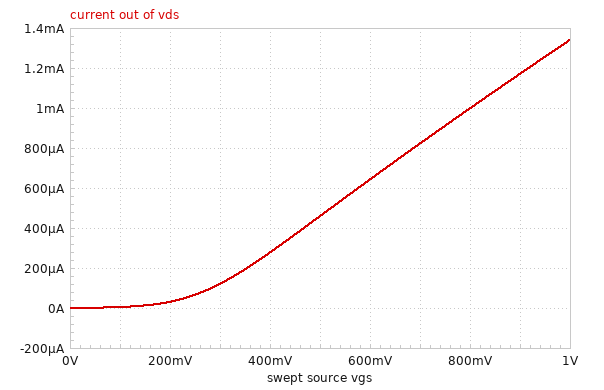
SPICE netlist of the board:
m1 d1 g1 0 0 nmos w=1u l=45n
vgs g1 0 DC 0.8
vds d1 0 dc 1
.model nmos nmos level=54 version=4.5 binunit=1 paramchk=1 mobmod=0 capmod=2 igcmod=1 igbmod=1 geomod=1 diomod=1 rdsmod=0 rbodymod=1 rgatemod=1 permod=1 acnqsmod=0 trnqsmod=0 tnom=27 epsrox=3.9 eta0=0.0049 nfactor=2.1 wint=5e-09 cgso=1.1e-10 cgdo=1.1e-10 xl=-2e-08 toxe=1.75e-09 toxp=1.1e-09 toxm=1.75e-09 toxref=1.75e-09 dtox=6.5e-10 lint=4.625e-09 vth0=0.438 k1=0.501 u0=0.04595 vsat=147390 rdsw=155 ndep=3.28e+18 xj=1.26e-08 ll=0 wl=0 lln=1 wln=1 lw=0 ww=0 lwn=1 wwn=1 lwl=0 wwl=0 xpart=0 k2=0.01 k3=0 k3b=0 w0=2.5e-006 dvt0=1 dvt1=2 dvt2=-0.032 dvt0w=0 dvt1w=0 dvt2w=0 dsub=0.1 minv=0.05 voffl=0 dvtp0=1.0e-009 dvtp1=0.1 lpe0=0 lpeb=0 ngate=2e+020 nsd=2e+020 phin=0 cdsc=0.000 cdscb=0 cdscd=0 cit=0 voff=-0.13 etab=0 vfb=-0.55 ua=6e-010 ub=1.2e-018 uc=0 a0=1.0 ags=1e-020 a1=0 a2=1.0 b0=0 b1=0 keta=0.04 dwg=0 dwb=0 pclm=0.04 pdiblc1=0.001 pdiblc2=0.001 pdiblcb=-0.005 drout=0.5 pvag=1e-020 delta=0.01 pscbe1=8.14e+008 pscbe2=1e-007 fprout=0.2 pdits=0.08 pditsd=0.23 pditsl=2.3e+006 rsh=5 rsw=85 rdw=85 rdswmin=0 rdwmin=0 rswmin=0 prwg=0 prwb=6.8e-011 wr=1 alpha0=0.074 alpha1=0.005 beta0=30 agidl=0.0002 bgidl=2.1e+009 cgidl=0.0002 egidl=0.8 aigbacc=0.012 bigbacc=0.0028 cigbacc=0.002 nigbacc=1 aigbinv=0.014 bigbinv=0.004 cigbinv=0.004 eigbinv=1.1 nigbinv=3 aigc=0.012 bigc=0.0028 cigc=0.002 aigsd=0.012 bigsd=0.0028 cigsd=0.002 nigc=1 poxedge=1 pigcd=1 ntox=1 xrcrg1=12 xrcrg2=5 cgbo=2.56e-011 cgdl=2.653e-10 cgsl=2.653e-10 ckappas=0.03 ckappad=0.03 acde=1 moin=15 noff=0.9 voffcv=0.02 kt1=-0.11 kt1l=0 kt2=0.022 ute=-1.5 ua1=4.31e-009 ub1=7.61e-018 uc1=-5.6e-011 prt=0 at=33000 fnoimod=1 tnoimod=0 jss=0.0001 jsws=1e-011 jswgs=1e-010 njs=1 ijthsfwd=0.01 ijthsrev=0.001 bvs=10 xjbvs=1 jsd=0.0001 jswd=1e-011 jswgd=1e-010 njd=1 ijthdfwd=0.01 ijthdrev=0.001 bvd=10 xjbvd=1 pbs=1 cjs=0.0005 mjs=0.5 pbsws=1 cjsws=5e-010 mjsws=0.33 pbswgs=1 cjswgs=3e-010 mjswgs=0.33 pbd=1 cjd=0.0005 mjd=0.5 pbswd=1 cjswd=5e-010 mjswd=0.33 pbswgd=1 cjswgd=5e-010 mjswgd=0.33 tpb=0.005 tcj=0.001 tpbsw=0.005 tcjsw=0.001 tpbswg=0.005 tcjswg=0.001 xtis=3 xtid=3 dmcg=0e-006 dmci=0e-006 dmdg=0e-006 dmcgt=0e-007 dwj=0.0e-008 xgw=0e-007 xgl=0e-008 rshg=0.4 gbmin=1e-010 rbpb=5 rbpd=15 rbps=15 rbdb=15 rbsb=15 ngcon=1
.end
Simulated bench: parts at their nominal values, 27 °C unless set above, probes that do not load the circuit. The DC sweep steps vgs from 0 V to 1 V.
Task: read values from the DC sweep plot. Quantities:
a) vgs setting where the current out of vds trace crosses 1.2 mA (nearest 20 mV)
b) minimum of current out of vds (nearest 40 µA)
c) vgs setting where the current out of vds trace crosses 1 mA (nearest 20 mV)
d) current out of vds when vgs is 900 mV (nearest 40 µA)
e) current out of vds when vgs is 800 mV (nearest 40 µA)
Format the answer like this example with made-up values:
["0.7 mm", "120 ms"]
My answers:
["920 mV", "0 A", "800 mV", "1.16 mA", "1.00 mA"]
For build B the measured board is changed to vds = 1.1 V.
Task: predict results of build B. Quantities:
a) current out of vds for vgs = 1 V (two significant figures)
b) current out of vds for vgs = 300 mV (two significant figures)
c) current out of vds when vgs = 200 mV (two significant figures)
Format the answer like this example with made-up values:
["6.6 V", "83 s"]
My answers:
["1.4 mA", "150 µA", "44 µA"]
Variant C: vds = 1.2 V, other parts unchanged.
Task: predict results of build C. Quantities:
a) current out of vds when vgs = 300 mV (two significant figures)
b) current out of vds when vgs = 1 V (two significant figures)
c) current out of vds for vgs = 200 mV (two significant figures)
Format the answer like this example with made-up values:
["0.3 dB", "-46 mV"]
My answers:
["180 µA", "1.4 mA", "60 µA"]
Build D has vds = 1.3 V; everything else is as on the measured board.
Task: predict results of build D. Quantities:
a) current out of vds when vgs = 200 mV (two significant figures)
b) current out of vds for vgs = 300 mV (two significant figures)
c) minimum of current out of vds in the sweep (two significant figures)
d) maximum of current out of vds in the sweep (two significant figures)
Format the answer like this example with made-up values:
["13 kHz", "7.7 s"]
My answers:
["81 µA", "220 µA", "2.3 µA", "1.5 mA"]
